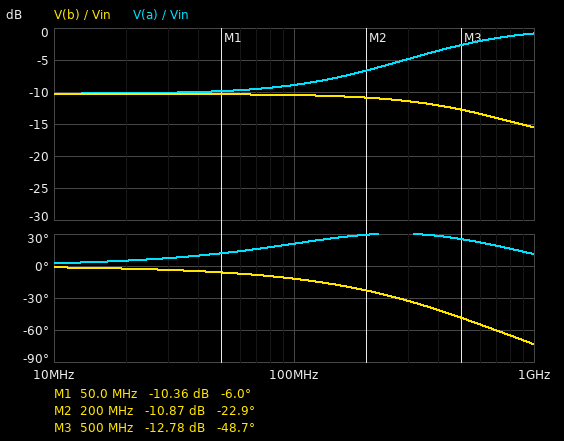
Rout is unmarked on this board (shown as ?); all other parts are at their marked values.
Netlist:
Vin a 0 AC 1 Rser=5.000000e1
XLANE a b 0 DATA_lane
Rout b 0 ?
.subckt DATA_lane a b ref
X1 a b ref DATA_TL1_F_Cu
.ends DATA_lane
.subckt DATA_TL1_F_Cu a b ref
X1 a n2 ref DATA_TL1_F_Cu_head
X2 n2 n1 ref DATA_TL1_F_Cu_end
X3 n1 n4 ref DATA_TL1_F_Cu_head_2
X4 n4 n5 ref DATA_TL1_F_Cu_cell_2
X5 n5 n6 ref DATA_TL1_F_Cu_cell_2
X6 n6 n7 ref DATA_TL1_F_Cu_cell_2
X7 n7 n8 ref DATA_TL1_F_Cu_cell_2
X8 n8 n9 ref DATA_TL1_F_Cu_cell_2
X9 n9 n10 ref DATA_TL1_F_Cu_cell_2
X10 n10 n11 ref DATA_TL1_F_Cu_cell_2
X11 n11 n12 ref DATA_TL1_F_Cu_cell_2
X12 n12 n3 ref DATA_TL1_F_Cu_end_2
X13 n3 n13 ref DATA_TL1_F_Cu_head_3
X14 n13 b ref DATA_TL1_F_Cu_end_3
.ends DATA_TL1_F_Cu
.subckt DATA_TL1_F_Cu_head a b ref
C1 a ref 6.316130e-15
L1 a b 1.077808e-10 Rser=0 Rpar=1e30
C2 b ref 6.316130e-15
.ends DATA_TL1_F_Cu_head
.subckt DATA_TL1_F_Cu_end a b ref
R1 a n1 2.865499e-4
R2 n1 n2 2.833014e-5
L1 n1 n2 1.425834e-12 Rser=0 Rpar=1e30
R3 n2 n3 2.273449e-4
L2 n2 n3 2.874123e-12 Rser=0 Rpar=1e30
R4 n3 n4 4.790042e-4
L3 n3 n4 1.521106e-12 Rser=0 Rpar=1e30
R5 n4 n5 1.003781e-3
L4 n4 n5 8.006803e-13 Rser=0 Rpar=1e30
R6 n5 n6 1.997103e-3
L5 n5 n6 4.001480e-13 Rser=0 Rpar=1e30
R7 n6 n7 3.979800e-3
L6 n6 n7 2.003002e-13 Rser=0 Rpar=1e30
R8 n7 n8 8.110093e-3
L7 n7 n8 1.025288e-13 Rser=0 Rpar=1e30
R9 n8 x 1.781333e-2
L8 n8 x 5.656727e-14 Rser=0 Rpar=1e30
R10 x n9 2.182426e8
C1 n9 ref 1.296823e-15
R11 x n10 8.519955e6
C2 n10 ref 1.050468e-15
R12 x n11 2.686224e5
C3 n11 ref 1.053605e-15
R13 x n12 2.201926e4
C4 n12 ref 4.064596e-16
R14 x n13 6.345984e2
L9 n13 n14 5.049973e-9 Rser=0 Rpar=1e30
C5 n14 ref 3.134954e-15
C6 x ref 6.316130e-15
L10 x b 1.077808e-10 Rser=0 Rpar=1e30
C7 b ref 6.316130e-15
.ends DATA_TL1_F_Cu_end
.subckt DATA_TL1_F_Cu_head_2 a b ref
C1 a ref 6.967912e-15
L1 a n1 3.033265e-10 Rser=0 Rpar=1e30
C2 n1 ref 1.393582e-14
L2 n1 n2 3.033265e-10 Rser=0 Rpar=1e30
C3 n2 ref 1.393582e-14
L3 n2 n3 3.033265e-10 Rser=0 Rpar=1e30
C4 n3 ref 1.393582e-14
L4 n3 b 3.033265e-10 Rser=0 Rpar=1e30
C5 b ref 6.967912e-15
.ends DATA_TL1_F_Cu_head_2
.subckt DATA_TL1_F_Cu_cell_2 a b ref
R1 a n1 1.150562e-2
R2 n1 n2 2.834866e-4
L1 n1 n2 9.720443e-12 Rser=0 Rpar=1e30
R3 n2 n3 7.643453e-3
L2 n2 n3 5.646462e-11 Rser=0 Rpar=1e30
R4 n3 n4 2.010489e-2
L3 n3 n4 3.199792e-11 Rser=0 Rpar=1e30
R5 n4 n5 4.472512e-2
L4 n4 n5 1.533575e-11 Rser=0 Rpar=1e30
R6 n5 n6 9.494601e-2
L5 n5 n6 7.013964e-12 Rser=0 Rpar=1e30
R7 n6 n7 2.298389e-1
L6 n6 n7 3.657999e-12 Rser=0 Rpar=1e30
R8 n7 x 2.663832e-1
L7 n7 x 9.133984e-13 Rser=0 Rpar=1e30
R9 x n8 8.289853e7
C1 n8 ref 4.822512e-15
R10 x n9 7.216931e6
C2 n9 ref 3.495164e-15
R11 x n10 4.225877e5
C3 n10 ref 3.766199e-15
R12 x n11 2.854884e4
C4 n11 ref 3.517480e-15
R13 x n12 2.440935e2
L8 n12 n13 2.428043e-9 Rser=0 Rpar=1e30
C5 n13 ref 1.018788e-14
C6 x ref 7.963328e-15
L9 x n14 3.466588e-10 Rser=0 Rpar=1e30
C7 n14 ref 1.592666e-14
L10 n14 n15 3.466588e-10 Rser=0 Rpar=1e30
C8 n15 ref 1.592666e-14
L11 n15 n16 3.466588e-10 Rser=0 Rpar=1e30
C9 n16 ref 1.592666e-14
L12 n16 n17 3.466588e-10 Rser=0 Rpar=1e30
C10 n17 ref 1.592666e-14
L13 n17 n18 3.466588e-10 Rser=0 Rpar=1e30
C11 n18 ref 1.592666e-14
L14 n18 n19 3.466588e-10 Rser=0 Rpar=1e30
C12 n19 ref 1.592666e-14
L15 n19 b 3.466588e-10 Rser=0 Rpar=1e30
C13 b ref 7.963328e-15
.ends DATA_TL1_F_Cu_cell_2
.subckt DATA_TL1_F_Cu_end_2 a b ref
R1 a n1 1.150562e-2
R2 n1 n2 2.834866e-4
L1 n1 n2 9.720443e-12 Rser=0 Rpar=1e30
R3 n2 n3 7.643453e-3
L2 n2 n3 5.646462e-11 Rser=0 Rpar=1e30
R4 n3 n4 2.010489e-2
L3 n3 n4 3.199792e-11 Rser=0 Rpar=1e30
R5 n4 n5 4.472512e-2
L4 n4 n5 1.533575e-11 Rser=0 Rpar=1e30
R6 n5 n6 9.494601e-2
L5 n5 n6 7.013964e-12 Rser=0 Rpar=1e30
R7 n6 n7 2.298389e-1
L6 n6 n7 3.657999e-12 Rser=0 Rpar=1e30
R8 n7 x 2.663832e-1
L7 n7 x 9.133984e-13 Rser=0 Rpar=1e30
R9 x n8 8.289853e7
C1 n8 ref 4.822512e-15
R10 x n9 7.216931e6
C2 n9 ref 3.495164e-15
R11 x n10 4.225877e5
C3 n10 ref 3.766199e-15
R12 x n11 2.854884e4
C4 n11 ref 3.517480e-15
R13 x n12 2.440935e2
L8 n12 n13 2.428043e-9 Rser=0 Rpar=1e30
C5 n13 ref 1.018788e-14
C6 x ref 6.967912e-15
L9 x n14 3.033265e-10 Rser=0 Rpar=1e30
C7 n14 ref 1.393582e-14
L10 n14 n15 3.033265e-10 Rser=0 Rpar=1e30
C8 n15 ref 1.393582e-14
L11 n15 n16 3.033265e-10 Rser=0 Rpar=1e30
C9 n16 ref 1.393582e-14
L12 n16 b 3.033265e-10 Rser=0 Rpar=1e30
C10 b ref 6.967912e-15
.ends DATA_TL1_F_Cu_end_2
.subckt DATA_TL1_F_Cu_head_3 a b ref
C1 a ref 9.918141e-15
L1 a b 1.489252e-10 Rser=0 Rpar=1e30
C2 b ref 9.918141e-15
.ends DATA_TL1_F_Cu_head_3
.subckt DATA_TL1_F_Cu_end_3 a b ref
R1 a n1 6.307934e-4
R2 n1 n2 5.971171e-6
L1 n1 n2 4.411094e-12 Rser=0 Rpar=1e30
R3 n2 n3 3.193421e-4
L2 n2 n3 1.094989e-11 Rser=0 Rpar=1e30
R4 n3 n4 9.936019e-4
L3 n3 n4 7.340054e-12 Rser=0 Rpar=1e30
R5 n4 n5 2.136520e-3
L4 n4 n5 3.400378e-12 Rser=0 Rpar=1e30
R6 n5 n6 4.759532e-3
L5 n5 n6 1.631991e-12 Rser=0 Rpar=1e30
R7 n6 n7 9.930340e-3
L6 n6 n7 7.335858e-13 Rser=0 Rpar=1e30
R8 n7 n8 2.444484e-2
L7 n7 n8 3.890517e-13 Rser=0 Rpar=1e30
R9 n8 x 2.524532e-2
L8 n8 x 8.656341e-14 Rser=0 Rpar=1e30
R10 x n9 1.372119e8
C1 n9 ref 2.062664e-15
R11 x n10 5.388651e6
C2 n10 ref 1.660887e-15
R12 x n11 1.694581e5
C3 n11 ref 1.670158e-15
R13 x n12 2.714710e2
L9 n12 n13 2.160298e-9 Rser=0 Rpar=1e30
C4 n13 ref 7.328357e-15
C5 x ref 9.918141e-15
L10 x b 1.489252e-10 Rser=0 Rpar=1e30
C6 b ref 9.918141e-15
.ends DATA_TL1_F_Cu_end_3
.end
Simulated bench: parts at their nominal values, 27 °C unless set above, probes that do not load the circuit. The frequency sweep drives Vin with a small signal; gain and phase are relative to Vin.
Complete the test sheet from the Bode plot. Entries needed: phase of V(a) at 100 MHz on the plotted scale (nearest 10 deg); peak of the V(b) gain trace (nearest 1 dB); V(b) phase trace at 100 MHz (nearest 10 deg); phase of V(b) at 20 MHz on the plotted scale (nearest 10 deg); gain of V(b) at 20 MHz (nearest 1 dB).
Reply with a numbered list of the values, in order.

1. 20 deg
2. -10 dB
3. -10 deg
4. 0 deg
5. -10 dB
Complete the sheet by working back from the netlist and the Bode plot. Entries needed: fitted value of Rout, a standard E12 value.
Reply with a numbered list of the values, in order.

1. 22 Ω
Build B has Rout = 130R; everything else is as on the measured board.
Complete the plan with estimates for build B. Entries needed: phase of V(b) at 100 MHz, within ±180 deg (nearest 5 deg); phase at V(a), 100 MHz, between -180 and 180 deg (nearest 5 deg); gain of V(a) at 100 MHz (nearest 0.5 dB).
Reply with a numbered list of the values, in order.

1. -5 deg
2. 0 deg
3. -3.0 dB
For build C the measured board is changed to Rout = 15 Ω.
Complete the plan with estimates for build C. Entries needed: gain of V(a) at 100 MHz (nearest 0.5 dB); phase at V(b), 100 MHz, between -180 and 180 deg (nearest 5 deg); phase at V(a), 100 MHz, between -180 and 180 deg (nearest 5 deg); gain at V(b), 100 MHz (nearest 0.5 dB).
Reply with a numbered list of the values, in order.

1. -10.0 dB
2. -15 deg
3. 30 deg
4. -13.0 dB
